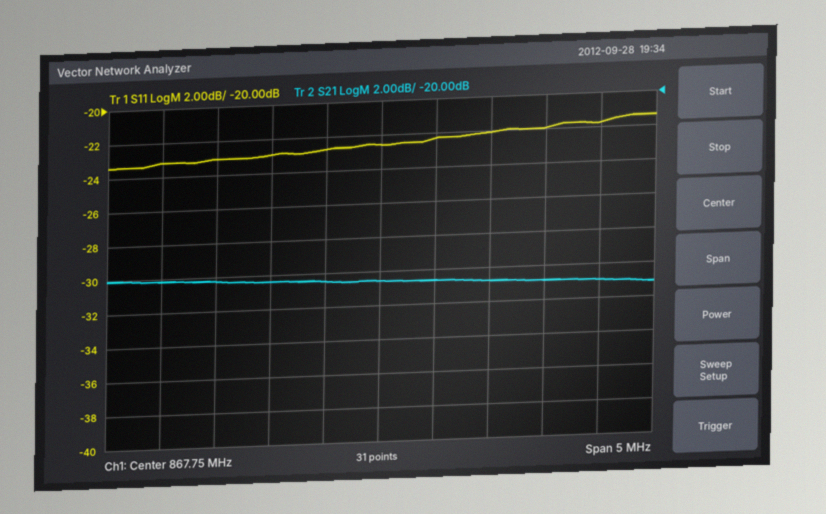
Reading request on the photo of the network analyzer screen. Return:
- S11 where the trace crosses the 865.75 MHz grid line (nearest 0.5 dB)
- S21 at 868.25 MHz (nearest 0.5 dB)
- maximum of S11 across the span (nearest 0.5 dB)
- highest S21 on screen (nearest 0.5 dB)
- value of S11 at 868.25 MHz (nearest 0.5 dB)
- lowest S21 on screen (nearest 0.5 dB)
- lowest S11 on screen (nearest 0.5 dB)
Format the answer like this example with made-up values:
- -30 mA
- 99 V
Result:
- -23.0 dB
- -30.5 dB
- -21.5 dB
- -30.0 dB
- -22.5 dB
- -31.0 dB
- -23.5 dB
